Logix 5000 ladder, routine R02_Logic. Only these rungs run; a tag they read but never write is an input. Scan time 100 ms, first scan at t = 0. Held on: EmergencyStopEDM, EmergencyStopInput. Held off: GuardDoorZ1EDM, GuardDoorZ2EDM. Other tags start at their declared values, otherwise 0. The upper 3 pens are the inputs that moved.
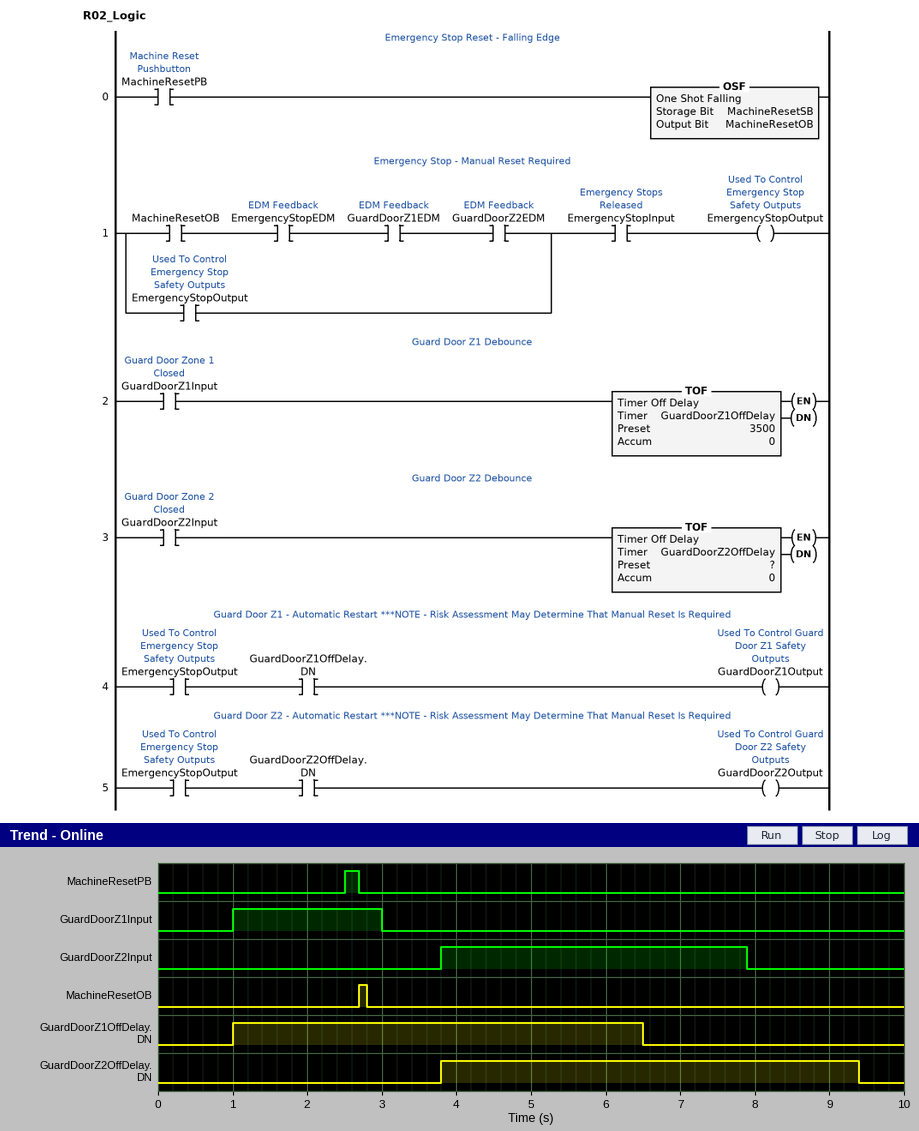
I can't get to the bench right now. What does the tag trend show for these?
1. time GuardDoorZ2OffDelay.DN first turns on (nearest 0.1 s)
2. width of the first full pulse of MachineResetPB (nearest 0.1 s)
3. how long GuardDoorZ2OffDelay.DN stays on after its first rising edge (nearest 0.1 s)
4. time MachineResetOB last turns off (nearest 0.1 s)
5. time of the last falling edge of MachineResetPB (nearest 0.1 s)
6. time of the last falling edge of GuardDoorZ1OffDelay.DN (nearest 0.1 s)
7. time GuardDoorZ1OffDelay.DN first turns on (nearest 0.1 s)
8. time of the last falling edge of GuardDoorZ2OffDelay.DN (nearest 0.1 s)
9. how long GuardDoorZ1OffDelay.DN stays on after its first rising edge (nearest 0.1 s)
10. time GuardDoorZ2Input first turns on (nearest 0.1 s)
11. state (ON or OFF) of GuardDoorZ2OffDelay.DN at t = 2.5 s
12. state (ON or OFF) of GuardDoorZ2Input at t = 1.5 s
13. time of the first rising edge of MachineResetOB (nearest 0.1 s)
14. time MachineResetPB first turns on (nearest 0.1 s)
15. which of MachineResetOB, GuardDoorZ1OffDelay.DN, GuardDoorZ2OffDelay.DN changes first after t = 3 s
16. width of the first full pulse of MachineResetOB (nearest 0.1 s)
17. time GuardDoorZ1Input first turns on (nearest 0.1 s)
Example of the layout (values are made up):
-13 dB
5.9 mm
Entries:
3.8 s
0.2 s
5.6 s
2.8 s
2.7 s
6.5 s
1.0 s
9.4 s
5.5 s
3.8 s
OFF
OFF
2.7 s
2.5 s
GuardDoorZ2OffDelay.DN
0.1 s
1.0 s
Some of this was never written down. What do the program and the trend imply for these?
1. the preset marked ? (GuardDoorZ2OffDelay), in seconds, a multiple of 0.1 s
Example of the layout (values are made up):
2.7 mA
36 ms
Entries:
1.5 s
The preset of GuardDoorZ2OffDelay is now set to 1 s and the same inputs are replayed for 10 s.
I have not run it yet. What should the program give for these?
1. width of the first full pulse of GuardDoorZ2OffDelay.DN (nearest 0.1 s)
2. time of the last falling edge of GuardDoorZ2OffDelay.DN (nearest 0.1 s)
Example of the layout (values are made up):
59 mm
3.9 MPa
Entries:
5.1 s
8.9 s
